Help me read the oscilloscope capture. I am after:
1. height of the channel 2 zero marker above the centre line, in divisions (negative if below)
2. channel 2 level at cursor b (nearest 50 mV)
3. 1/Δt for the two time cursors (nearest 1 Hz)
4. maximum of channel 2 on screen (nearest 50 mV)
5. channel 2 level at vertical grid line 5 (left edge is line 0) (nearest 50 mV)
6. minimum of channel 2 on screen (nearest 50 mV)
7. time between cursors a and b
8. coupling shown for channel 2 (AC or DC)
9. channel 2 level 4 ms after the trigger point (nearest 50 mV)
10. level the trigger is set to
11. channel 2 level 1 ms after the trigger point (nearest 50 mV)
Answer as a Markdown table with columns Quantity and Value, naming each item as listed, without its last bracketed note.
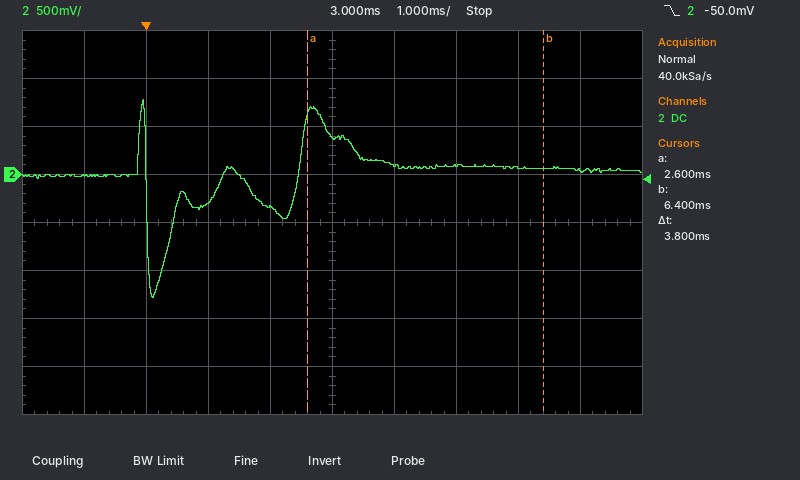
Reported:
| Quantity | Value |
|---|---|
| height of the channel 2 zero marker above the centre line, in divisions | +1.0 div |
| channel 2 level at cursor b | 50 mV |
| 1/Δt for the two time cursors | 263 Hz |
| maximum of channel 2 on screen | 800 mV |
| channel 2 level at vertical grid line 5 (left edge is line 0) | 400 mV |
| minimum of channel 2 on screen | -1.30 V |
| time between cursors a and b | 3.8 ms |
| coupling shown for channel 2 | DC |
| channel 2 level 4 ms after the trigger point | 100 mV |
| level the trigger is set to | -50.0 mV |
| channel 2 level 1 ms after the trigger point | -300 mV |
